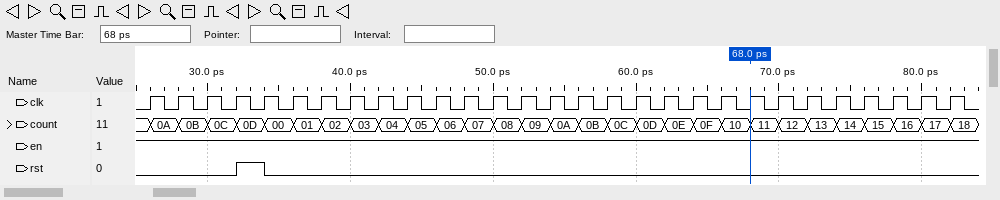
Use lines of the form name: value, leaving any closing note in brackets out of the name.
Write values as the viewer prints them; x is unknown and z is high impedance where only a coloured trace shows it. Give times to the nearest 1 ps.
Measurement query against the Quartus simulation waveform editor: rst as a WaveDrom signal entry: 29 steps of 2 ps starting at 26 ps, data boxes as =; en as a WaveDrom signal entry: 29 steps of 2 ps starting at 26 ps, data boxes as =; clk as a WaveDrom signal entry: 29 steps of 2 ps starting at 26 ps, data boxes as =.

rst as a WaveDrom signal entry: 29 steps of 2 ps starting at 26 ps, data boxes as =: {name: 'rst', wave: '0..10........................'}
en as a WaveDrom signal entry: 29 steps of 2 ps starting at 26 ps, data boxes as =: {name: 'en', wave: '1............................'}
clk as a WaveDrom signal entry: 29 steps of 2 ps starting at 26 ps, data boxes as =: {name: 'clk', wave: 'p............................'}
